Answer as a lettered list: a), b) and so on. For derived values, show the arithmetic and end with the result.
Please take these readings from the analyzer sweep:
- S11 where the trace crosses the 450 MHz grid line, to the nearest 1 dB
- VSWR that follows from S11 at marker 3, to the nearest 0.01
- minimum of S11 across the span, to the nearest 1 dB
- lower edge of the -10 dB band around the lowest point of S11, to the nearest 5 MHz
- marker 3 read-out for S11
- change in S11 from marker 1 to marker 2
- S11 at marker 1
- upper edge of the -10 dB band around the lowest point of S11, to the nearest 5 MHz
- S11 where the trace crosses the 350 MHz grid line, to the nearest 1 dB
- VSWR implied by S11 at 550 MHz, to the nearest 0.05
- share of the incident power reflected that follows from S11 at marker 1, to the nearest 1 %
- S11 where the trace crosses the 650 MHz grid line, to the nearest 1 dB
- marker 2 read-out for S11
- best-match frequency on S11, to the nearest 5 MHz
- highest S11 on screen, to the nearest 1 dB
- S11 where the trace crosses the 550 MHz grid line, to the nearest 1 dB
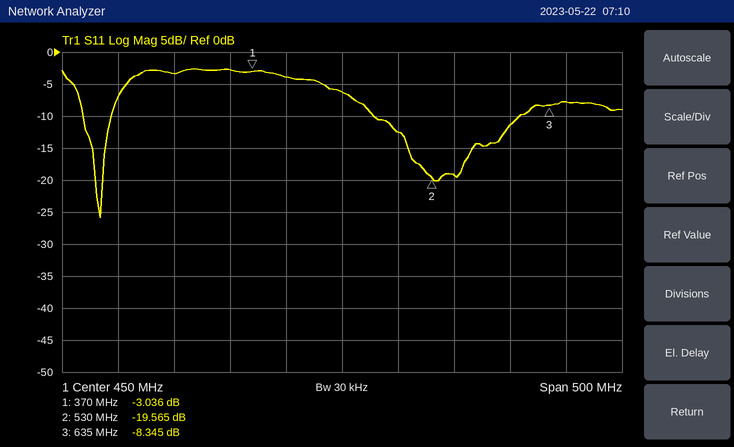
a) -6 dB
b) (1 + 0.3826)/(1 − 0.3826) ≈ 2.24
c) -26 dB
d) 220 MHz
e) -8.345 dB
f) -19.565 − (-3.036) = -16.529 dB
g) -3.036 dB
h) 245 MHz
i) -3 dB
j) |Γ| = 10^(-19/20) = 0.1122; VSWR = (1 + 0.1122)/(1 − 0.1122) ≈ 1.25
k) 10^(-3.036/10) ≈ 50 %
l) -8 dB
m) -19.565 dB
n) 235 MHz
o) -3 dB
p) -19 dB
